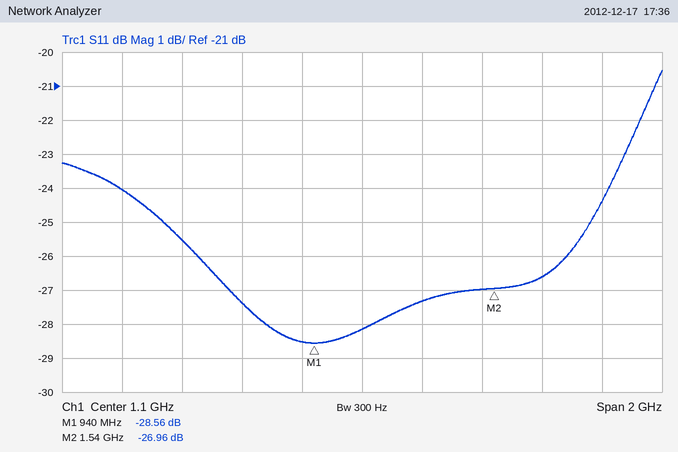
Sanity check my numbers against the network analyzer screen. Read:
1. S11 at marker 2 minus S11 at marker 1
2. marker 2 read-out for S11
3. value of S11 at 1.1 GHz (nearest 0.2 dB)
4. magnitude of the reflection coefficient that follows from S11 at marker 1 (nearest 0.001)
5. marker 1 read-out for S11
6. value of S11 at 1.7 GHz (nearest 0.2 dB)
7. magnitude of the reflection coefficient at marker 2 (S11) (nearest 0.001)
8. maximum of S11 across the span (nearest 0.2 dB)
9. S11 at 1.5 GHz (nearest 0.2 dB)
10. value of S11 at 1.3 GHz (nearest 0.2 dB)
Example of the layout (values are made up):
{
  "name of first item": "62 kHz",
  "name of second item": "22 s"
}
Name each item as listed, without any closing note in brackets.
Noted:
{
  "S11 at marker 2 minus S11 at marker 1": "1.60 dB",
  "marker 2 read-out for S11": "-26.96 dB",
  "value of S11 at 1.1 GHz": "-28.2 dB",
  "magnitude of the reflection coefficient that follows from S11 at marker 1": "0.037",
  "marker 1 read-out for S11": "-28.56 dB",
  "value of S11 at 1.7 GHz": "-26.6 dB",
  "magnitude of the reflection coefficient at marker 2 (S11)": "0.045",
  "maximum of S11 across the span": "-20.6 dB",
  "S11 at 1.5 GHz": "-27.0 dB",
  "value of S11 at 1.3 GHz": "-27.4 dB"
}
